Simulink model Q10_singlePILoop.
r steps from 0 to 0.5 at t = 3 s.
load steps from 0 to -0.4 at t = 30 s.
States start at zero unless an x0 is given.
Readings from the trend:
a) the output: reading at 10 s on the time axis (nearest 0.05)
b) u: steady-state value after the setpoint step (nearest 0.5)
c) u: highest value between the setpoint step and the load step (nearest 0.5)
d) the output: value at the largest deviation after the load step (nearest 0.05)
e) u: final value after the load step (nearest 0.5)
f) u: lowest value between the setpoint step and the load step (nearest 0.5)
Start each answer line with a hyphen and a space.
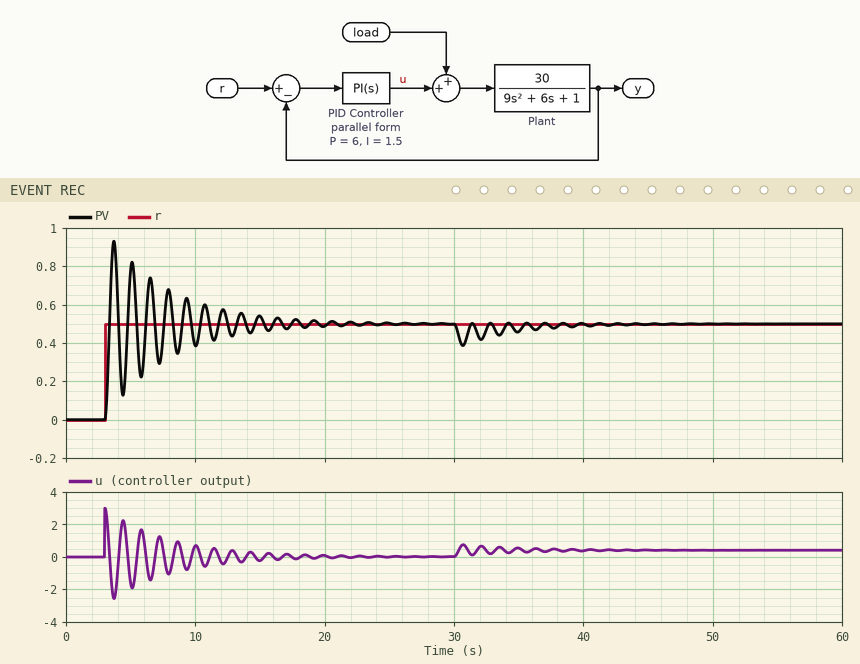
- 0.40
- 0.0
- 3.0
- 0.40
- 0.5
- -2.5
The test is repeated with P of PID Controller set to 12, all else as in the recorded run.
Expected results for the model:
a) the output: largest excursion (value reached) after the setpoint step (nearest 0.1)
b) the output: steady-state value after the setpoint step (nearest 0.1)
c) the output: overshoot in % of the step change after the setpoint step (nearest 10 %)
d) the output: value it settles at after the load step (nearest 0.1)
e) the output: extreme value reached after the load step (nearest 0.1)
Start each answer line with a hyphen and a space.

- 0.9
- 0.5
- 90 %
- 0.5
- 0.4
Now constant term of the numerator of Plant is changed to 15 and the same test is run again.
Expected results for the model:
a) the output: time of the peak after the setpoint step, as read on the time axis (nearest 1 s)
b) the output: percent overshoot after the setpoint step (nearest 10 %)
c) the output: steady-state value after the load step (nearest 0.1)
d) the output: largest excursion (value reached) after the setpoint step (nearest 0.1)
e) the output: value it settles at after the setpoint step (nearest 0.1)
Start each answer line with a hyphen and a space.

- 4 s
- 80 %
- 0.5
- 0.9
- 0.5
